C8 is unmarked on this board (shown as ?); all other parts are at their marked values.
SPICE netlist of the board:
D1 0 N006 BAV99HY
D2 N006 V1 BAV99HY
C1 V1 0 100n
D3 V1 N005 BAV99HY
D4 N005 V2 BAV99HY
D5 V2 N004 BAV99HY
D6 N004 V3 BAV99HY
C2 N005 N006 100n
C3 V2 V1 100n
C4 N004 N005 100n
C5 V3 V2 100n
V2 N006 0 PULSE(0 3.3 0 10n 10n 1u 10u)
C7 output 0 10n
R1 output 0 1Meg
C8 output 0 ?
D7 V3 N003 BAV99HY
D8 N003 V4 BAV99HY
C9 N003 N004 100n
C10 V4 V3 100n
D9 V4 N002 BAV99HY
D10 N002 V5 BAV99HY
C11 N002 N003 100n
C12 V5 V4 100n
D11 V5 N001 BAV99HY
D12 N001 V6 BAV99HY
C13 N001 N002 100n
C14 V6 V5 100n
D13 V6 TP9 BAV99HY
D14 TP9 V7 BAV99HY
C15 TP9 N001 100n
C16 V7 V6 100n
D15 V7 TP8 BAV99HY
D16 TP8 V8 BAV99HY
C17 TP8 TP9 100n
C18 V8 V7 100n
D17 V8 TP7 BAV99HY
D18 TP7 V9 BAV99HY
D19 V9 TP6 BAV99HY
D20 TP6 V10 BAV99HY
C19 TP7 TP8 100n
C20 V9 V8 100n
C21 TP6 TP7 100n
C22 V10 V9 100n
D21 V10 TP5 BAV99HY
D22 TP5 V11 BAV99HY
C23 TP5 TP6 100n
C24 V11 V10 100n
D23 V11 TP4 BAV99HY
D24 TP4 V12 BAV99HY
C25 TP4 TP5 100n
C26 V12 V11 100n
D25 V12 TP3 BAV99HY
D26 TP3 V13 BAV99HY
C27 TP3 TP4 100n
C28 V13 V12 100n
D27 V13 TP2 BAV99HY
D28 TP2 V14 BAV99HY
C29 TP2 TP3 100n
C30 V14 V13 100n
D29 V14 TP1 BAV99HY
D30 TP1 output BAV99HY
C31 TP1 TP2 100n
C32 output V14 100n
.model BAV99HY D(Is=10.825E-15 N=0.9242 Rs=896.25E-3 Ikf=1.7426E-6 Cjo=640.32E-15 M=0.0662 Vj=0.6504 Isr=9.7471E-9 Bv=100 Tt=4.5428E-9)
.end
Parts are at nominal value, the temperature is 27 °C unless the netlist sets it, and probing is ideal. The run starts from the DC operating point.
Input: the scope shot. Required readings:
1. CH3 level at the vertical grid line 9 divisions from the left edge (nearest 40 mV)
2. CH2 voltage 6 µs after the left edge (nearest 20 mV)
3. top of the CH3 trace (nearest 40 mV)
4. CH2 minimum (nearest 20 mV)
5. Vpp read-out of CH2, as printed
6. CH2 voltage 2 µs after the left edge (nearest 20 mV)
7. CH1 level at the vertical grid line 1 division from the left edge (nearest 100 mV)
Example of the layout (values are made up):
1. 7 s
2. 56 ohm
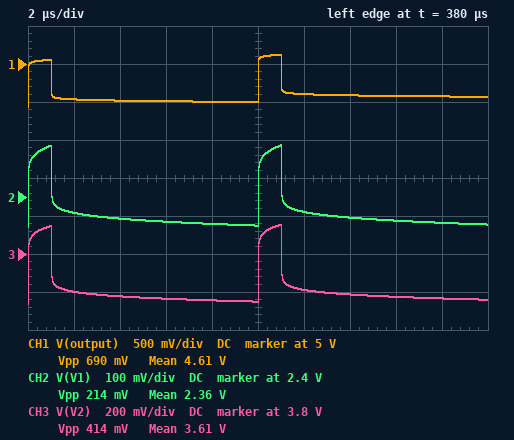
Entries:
1. 3.56 V
2. 2.34 V
3. 3.96 V
4. 2.32 V
5. 214 mV
6. 2.36 V
7. 4.5 V
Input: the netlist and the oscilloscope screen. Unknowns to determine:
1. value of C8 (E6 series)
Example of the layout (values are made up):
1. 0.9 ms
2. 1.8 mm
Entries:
1. 6.8 nF
